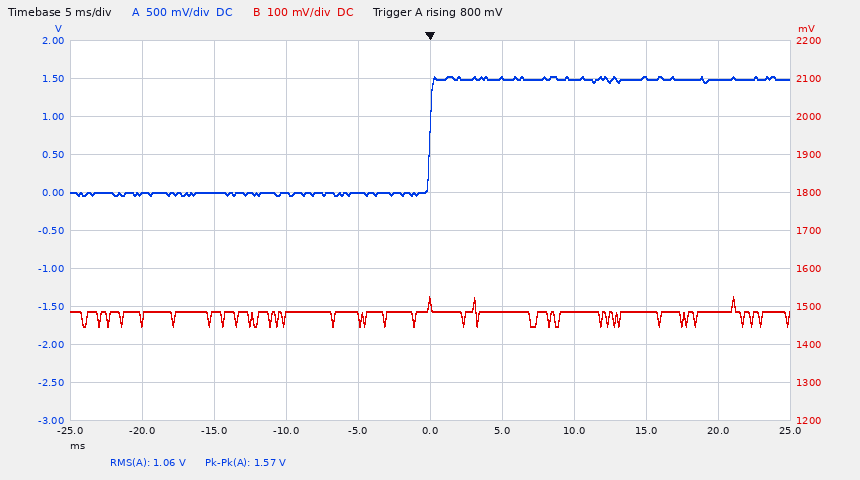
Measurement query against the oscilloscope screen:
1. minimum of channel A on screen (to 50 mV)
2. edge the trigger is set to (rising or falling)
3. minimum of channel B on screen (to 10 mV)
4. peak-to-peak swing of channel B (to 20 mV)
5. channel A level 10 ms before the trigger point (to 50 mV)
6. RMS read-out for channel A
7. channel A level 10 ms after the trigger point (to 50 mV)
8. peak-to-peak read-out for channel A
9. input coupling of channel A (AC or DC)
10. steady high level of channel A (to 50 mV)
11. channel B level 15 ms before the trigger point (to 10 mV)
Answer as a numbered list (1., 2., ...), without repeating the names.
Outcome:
1. -50 mV
2. rising
3. 1.45 V
4. 80 mV
5. 0 mV
6. 1.06 V
7. 1.50 V
8. 1.57 V
9. DC
10. 1.50 V
11. 1.48 V
